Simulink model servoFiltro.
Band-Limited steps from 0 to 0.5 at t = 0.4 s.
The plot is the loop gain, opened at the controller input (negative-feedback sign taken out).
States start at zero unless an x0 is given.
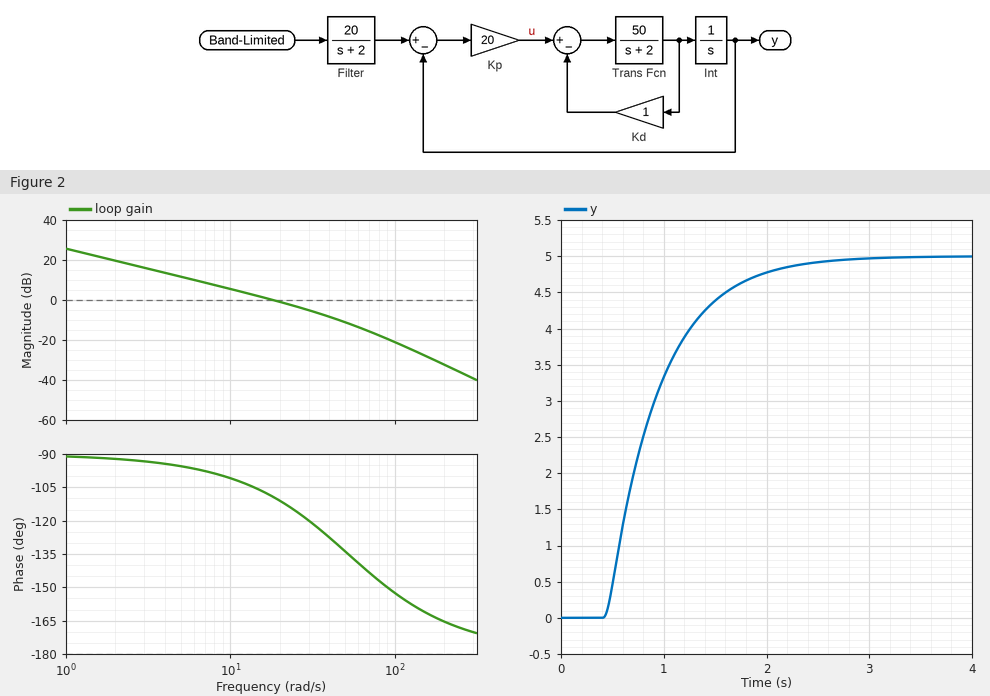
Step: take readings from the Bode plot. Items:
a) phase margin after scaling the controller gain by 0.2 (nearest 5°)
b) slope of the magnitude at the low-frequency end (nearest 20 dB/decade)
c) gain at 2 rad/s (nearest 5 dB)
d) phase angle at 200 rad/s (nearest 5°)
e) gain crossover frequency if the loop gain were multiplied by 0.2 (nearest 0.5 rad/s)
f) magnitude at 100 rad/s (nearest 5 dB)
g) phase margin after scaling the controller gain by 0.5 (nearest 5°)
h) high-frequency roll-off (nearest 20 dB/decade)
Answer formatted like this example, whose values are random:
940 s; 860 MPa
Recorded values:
85°; -20 dB/decade; 20 dB; -165°; 4.0 rad/s; -20 dB; 80°; -40 dB/decade
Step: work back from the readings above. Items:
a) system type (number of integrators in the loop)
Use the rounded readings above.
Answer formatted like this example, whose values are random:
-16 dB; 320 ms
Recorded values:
1
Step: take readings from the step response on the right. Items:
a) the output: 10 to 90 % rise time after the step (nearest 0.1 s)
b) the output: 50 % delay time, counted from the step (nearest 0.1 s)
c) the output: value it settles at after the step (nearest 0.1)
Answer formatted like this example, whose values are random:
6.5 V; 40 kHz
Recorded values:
1.1 s; 0.4 s; 5.0
